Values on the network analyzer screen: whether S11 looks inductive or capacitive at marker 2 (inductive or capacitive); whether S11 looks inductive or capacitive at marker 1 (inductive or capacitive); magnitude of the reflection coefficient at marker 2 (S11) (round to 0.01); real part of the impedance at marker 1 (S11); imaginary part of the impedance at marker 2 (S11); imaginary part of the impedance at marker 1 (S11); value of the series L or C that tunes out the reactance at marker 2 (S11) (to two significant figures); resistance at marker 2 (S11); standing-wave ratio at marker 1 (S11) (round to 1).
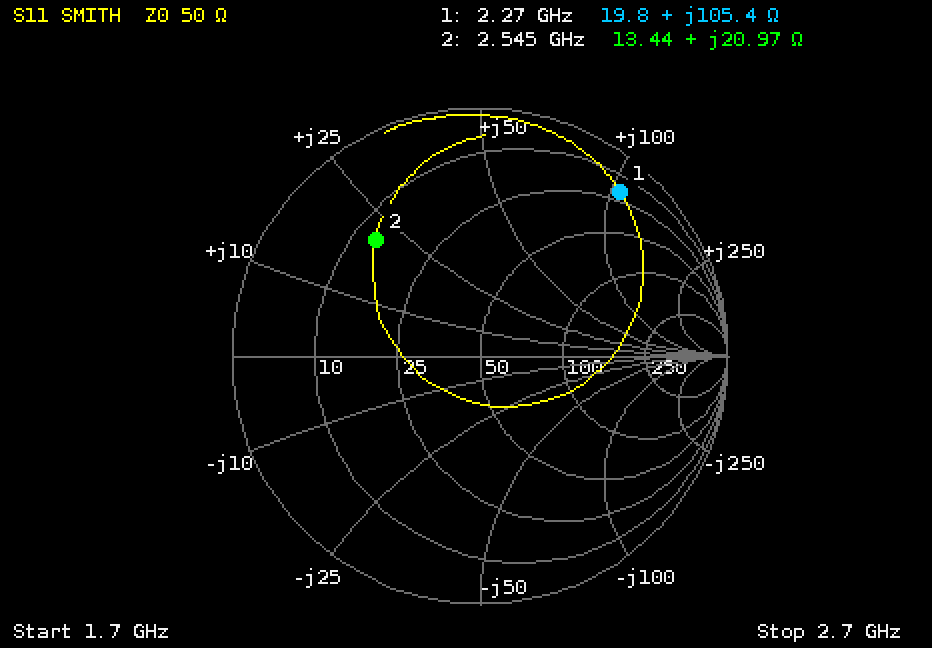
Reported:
inductive
inductive
0.63
19.8 Ω
+20.97 Ω
+105.4 Ω
3.0 pF
13.44 Ω
14
